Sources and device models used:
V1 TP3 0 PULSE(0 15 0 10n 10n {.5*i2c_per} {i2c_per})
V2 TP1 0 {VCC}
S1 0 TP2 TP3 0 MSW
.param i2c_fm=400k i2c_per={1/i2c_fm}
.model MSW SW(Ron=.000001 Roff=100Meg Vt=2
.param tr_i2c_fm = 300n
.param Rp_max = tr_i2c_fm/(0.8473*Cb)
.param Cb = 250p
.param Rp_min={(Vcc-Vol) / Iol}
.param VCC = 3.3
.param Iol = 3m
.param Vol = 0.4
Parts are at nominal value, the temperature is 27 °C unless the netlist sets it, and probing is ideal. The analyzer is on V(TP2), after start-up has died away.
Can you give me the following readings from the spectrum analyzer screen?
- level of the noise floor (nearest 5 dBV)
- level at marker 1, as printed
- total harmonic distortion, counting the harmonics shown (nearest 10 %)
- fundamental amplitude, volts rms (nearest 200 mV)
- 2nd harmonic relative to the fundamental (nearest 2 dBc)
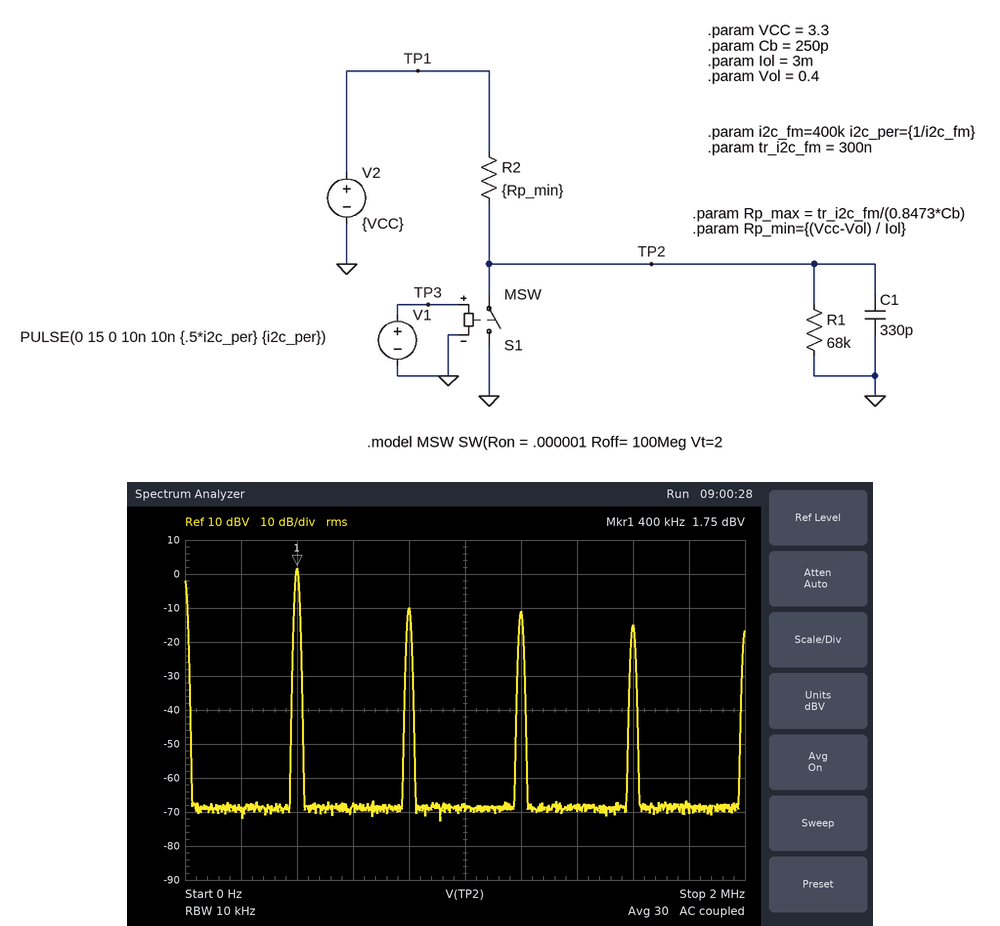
-70 dBV
1.75 dBV
40 %
1.2 V
-12 dBc
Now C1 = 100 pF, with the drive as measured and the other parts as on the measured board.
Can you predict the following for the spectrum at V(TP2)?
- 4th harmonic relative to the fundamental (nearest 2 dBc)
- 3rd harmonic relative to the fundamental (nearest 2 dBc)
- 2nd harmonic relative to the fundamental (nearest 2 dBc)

-20 dBc
-10 dBc
-18 dBc
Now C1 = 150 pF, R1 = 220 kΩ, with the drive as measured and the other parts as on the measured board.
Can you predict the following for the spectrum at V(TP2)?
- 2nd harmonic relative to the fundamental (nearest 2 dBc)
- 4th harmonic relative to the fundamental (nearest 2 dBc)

-16 dBc
-18 dBc
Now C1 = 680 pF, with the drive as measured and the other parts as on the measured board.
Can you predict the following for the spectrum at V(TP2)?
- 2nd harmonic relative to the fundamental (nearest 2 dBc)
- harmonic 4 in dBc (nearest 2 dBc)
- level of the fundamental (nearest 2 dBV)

-10 dBc
-16 dBc
0 dBV
